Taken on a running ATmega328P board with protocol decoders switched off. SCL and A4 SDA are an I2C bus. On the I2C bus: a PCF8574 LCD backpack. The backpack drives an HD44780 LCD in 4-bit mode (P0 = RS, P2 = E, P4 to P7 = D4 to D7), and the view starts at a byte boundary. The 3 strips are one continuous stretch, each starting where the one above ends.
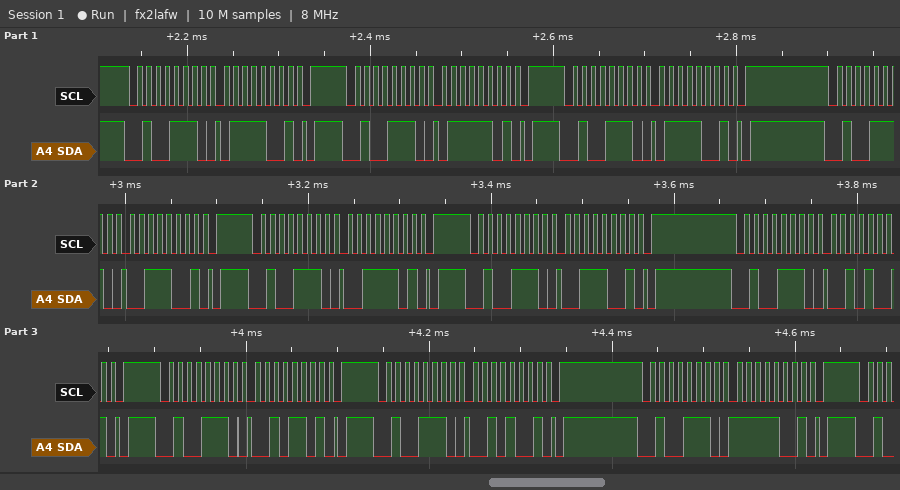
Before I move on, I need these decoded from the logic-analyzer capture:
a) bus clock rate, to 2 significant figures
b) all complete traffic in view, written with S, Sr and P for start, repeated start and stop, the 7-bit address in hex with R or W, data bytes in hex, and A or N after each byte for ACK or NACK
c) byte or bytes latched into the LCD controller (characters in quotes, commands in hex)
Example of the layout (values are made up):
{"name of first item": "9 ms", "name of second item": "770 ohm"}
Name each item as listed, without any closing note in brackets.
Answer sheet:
{"bus clock rate, to 2 significant figures": "100 kHz", "all complete traffic in view, written with S, Sr and P for start, repeated start and stop, the 7-bit address in hex with R or W, data bytes in hex, and A or N after each byte for ACK or NACK": "S 27W A 79 A P S 27W A 7D A P S 27W A 79 A P S 27W A 39 A P S 27W A 3D A P S 27W A 39 A P S 27W A 29 A P S 27W A 2D A P S 27W A 29 A P S 27W A F9 A P", "byte or bytes latched into the LCD controller": "'s'"}
